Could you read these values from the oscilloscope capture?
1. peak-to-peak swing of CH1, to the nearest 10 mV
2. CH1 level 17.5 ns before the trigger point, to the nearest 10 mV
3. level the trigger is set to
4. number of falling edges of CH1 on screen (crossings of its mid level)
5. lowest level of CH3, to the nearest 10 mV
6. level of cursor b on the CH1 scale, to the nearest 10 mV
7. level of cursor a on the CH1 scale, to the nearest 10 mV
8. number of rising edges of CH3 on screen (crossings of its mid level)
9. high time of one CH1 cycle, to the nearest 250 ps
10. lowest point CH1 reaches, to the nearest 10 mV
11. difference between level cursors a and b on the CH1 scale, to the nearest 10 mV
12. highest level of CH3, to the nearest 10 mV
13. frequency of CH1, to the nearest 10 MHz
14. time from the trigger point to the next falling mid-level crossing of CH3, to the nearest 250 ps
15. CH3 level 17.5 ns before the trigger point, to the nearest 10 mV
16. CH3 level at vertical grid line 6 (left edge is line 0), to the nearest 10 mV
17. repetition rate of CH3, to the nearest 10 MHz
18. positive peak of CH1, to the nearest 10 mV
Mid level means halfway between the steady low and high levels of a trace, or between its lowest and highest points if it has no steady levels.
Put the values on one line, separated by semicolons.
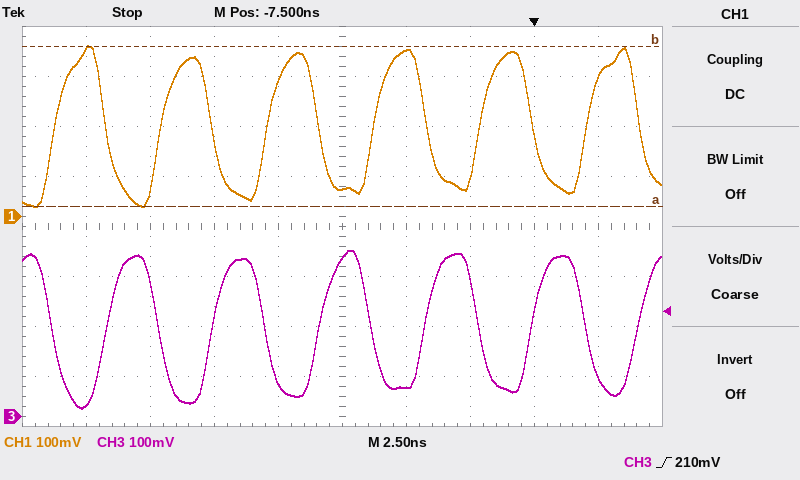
320 mV; 330 mV; 210 mV; 6; 20 mV; 340 mV; 20 mV; 6; 2.00 ns; 20 mV; 320 mV; 330 mV; 240 MHz; 2.00 ns; 20 mV; 60 mV; 240 MHz; 340 mV
